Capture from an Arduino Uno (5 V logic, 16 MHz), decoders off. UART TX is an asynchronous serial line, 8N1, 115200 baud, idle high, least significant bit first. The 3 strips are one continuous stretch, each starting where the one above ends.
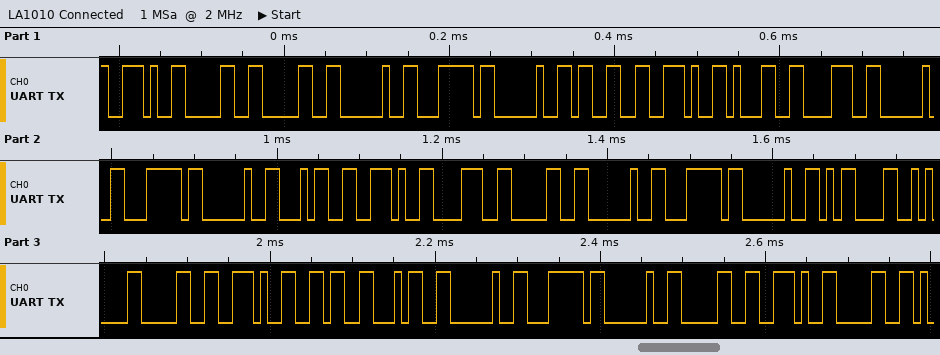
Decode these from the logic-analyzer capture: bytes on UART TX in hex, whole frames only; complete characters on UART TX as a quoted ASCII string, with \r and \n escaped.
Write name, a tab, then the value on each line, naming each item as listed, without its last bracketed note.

bytes on UART TX in hex, whole frames only	2E 30 30 20 7C 20 33 2E 31 38 20 7C 20 34 2E 38 30 20 7C 20 0D 0A 30 2E 36 34 20 7C 20 30 2E 30
complete characters on UART TX as a quoted ASCII string, with \r and \n escaped	".00 | 3.18 | 4.80 | \r\n0.64 | 0.0"
